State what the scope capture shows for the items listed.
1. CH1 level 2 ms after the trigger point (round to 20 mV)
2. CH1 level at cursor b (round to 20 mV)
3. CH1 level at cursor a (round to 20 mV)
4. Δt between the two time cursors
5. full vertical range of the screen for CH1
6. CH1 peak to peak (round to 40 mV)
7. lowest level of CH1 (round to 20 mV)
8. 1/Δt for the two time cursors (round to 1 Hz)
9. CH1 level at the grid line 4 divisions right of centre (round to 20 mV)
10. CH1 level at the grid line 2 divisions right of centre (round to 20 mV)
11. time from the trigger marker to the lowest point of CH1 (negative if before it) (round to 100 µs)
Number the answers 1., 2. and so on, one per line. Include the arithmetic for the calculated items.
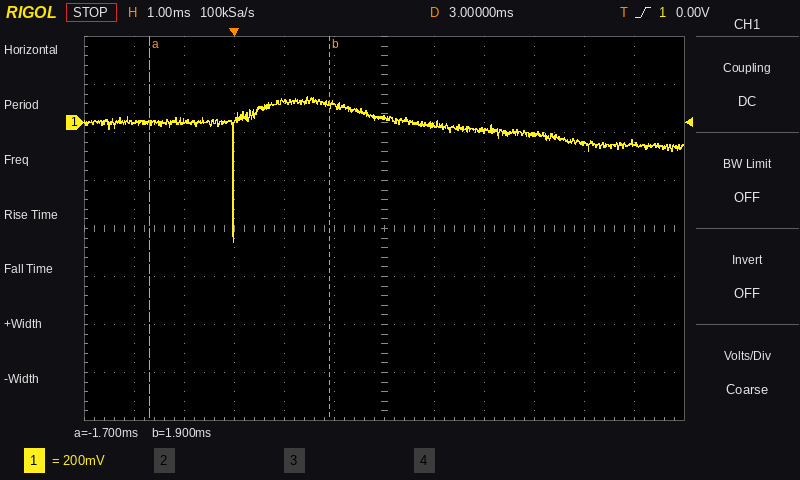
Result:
1. 80 mV
2. 80 mV
3. 0 mV
4. 1.9 ms − (-1.7 ms) = 3.6 ms
5. 1.6 V
6. 600 mV
7. -500 mV
8. 1 / 3.6 ms ≈ 278 Hz
9. -80 mV
10. -40 mV
11. 0.0 ms
